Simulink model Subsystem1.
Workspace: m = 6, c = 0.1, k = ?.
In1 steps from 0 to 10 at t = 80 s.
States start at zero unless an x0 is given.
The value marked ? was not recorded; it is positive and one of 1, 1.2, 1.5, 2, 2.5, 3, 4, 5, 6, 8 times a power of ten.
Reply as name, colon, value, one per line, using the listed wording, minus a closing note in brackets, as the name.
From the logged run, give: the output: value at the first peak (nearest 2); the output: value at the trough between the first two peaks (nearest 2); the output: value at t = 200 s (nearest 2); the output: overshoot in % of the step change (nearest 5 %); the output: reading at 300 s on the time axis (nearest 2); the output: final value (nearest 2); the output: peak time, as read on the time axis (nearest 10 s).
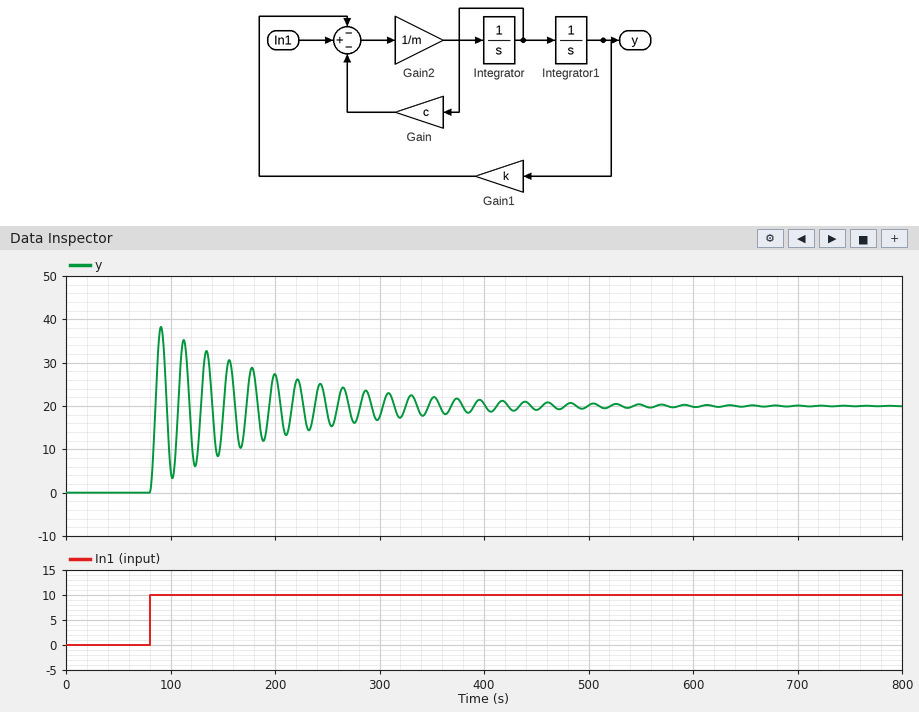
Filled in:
the output: value at the first peak: 38
the output: value at the trough between the first two peaks: 4
the output: value at t = 200 s: 28
the output: overshoot in % of the step change: 90 %
the output: reading at 300 s on the time axis: 18
the output: final value: 20
the output: peak time, as read on the time axis: 90 s
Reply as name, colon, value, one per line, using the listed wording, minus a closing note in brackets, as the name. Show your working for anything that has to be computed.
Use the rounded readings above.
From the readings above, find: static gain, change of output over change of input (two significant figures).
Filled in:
static gain, change of output over change of input: (20 - 0) / (10 - 0) = 2.0
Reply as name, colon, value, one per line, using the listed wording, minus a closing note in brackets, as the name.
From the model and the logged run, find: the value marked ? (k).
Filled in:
the value marked ?: 0.5
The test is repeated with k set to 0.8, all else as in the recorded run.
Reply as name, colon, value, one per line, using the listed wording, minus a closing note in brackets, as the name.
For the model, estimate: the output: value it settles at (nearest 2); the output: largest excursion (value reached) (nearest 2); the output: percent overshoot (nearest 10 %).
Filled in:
the output: value it settles at: 12
the output: largest excursion (value reached): 24
the output: percent overshoot: 90 %
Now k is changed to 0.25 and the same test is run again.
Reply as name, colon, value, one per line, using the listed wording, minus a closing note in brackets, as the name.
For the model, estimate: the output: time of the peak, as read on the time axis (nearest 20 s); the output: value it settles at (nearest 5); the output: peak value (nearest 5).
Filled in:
the output: time of the peak, as read on the time axis: 100 s
the output: value it settles at: 40
the output: peak value: 75
